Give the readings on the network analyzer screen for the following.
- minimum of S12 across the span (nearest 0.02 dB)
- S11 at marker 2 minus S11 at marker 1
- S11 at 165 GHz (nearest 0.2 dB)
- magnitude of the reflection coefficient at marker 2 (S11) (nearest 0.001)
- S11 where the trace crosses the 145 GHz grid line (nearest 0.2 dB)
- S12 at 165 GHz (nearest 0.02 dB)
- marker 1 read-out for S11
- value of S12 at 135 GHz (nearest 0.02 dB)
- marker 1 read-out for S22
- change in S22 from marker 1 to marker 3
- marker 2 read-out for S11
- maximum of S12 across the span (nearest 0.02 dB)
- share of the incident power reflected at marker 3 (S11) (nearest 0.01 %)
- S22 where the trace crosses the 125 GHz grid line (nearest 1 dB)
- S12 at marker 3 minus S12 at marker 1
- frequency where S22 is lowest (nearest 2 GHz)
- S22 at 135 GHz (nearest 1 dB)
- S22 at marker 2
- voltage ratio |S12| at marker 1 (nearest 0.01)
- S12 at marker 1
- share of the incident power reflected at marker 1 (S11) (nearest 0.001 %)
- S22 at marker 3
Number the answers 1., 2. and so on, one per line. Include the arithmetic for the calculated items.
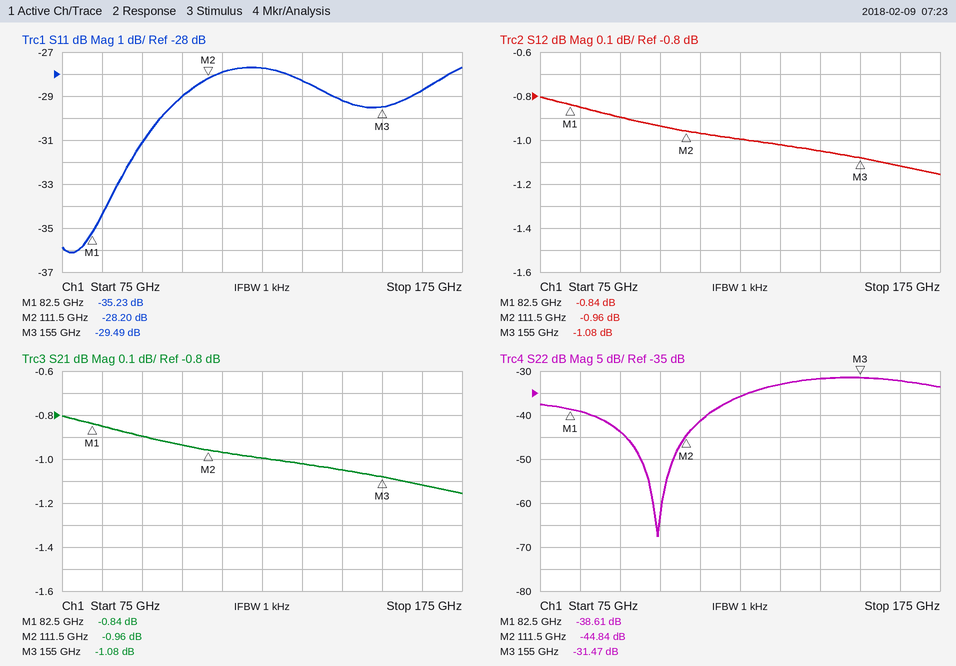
1. -1.16 dB
2. -28.2 − (-35.23) = 7.03 dB
3. -28.8 dB
4. 10^(-28.2/20) ≈ 0.039
5. -29.2 dB
6. -1.12 dB
7. -35.23 dB
8. -1.02 dB
9. -38.61 dB
10. -31.47 − (-38.61) = 7.14 dB
11. -28.20 dB
12. -0.80 dB
13. 10^(-29.49/10) ≈ 0.11 %
14. -36 dB
15. -1.08 − (-0.84) = -0.24 dB
16. 104 GHz
17. -33 dB
18. -44.84 dB
19. 10^(-0.84/20) ≈ 0.91
20. -0.84 dB
21. 10^(-35.23/10) ≈ 0.030 %
22. -31.47 dB
